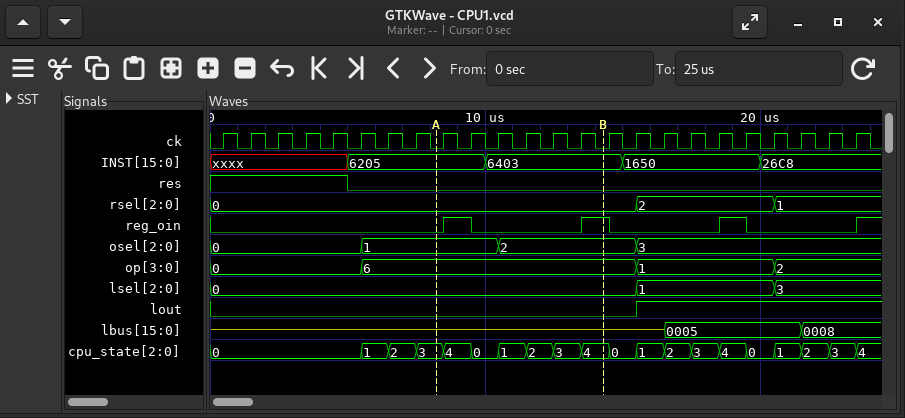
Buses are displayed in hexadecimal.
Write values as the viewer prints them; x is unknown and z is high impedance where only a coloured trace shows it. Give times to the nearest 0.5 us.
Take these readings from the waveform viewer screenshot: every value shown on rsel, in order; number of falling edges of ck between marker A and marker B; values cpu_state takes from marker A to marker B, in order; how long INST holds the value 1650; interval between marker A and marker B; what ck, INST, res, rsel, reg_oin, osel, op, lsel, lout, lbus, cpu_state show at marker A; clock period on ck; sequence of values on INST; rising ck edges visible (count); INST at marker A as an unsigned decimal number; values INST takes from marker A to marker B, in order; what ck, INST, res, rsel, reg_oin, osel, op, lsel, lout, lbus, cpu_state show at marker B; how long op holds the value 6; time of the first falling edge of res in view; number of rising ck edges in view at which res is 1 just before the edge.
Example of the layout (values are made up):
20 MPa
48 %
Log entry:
0, 2, 1
6
3, 4, 0, 1, 2, 3, 4
5 us
6 us
ck=0, INST=6205, res=0, rsel=0, reg_oin=0, osel=1, op=6, lsel=0, lout=0, lbus=z, cpu_state=3
1 us
xxxx, 6205, 6403, 1650, 26C8
24
25093
6205, 6403
ck=0, INST=6403, res=0, rsel=0, reg_oin=1, osel=2, op=6, lsel=0, lout=0, lbus=z, cpu_state=4
10 us
5 us
5
